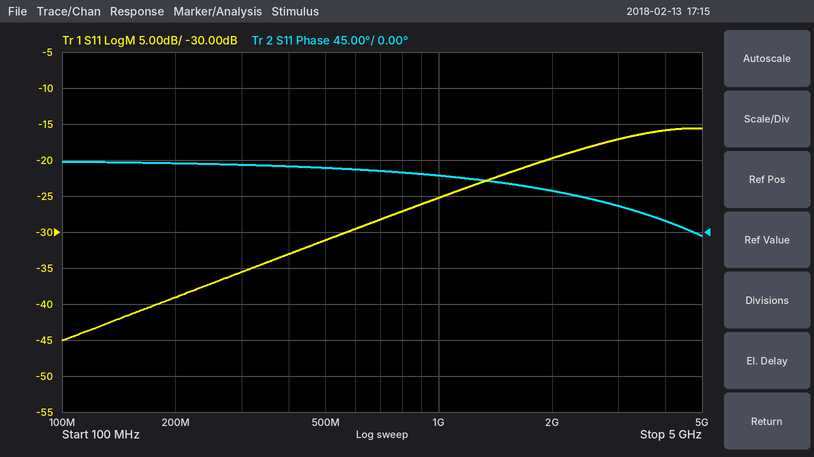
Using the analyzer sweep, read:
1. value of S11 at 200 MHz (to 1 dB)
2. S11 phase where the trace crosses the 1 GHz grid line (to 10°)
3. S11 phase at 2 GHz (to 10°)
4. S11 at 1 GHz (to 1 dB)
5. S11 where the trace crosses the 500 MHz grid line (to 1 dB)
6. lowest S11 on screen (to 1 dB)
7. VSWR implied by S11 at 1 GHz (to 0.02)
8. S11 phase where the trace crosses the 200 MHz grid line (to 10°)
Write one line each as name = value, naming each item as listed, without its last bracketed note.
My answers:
value of S11 at 200 MHz = -39 dB
S11 phase where the trace crosses the 1 GHz grid line = 70°
S11 phase at 2 GHz = 50°
S11 at 1 GHz = -25 dB
S11 where the trace crosses the 500 MHz grid line = -31 dB
lowest S11 on screen = -45 dB
VSWR implied by S11 at 1 GHz = 1.12
S11 phase where the trace crosses the 200 MHz grid line = 90°
